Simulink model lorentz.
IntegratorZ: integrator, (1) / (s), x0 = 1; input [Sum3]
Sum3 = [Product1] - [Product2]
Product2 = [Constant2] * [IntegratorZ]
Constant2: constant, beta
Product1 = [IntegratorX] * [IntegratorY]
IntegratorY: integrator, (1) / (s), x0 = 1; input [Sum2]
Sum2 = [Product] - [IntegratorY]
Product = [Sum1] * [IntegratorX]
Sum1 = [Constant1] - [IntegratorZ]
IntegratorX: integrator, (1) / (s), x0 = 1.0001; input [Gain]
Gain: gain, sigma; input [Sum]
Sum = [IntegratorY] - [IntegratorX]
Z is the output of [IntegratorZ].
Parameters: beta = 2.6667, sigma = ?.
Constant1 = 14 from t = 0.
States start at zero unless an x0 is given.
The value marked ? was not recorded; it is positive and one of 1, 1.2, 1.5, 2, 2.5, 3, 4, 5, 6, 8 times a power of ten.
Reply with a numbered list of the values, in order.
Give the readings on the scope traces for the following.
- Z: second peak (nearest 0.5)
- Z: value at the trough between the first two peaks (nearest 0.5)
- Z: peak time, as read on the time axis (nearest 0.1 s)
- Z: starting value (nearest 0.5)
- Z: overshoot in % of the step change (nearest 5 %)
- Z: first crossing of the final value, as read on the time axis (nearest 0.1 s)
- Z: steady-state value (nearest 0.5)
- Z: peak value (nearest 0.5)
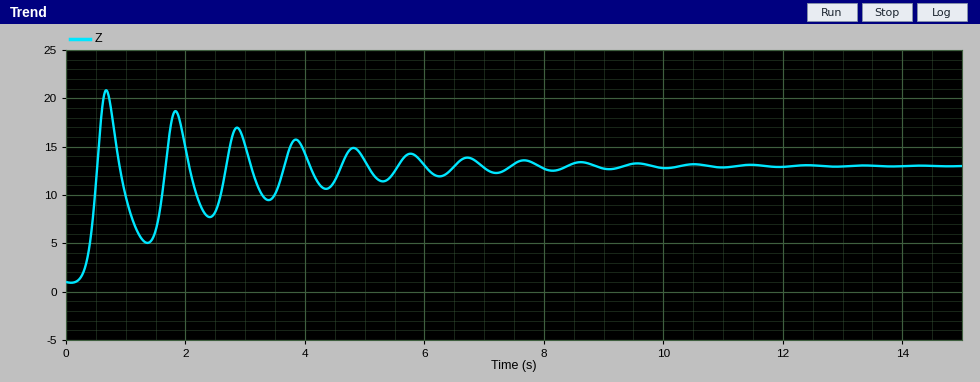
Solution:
1. 18.5
2. 5.0
3. 0.7 s
4. 1.0
5. 65 %
6. 0.5 s
7. 13.0
8. 21.0
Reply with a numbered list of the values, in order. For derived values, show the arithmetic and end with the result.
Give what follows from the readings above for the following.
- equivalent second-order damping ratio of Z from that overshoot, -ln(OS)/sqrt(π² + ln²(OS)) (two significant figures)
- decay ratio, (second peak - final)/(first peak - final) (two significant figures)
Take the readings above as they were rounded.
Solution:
1. ln(0.65) = -0.431; 0.431 / sqrt(9.870 + 0.186) = 0.14
2. (18.5 - 13) / (21 - 13) = 0.69
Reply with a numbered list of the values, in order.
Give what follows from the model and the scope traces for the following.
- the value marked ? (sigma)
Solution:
1. 5
